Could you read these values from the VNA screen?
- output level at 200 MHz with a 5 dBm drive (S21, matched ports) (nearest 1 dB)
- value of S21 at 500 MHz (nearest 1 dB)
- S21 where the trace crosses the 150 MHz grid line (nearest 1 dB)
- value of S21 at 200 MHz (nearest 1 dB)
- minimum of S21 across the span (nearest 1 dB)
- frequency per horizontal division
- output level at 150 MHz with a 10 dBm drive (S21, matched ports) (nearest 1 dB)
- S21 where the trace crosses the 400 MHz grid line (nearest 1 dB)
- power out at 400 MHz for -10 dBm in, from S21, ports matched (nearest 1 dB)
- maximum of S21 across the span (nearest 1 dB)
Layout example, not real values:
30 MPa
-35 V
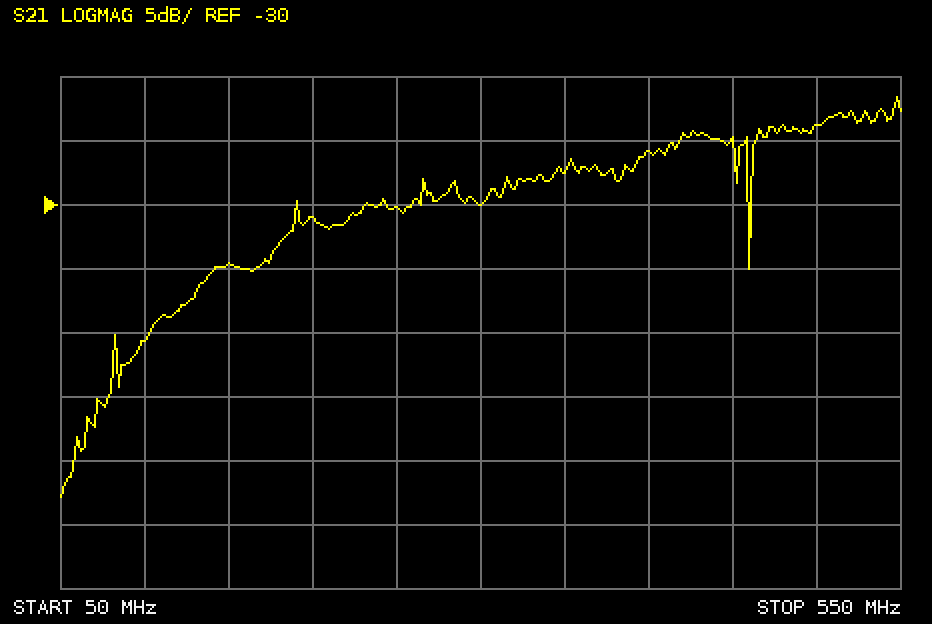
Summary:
-26 dBm
-24 dB
-35 dB
-31 dB
-53 dB
50 MHz
-25 dBm
-26 dB
-36 dBm
-22 dB
